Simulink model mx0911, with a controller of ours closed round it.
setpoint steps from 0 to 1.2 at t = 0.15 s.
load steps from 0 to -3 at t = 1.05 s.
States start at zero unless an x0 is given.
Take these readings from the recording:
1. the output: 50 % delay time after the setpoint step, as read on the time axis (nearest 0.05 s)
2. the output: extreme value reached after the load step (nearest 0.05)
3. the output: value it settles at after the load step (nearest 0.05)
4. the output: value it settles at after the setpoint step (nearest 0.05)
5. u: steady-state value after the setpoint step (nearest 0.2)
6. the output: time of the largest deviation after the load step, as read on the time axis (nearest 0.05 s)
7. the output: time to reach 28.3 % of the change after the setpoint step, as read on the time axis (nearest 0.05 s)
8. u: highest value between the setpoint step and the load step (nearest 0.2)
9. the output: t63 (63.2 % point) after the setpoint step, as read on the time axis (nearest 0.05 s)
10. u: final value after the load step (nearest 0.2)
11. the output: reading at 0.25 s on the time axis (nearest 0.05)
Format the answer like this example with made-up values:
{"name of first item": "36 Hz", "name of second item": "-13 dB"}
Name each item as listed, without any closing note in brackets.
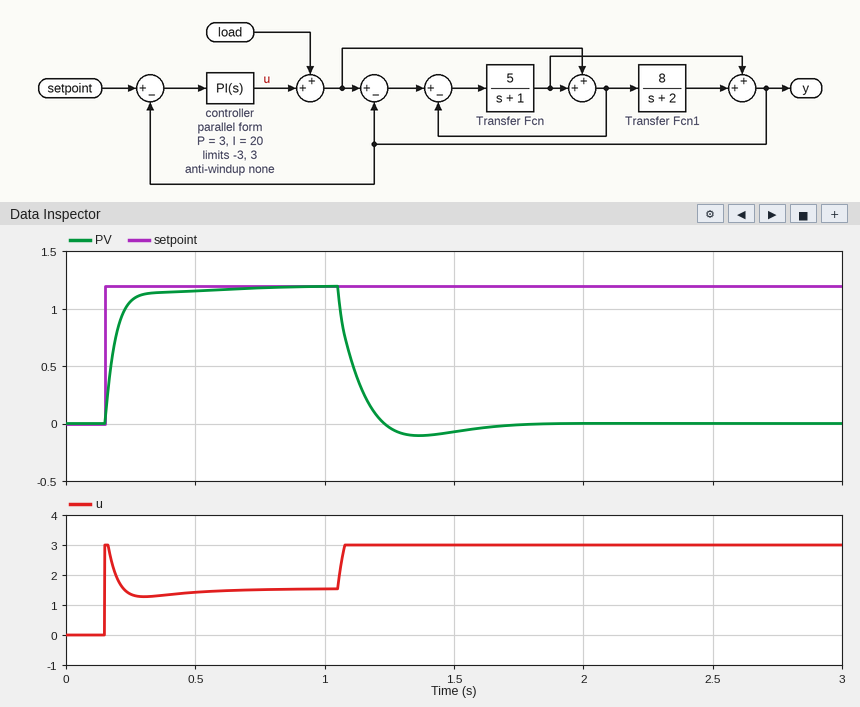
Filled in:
{"the output: 50 % delay time after the setpoint step, as read on the time axis": "0.20 s", "the output: extreme value reached after the load step": "-0.10", "the output: value it settles at after the load step": "0.00", "the output: value it settles at after the setpoint step": "1.20", "u: steady-state value after the setpoint step": "1.6", "the output: time of the largest deviation after the load step, as read on the time axis": "1.35 s", "the output: time to reach 28.3 % of the change after the setpoint step, as read on the time axis": "0.15 s", "u: highest value between the setpoint step and the load step": "3.0", "the output: t63 (63.2 % point) after the setpoint step, as read on the time axis": "0.20 s", "u: final value after the load step": "3.0", "the output: reading at 0.25 s on the time axis": "1.05"}
